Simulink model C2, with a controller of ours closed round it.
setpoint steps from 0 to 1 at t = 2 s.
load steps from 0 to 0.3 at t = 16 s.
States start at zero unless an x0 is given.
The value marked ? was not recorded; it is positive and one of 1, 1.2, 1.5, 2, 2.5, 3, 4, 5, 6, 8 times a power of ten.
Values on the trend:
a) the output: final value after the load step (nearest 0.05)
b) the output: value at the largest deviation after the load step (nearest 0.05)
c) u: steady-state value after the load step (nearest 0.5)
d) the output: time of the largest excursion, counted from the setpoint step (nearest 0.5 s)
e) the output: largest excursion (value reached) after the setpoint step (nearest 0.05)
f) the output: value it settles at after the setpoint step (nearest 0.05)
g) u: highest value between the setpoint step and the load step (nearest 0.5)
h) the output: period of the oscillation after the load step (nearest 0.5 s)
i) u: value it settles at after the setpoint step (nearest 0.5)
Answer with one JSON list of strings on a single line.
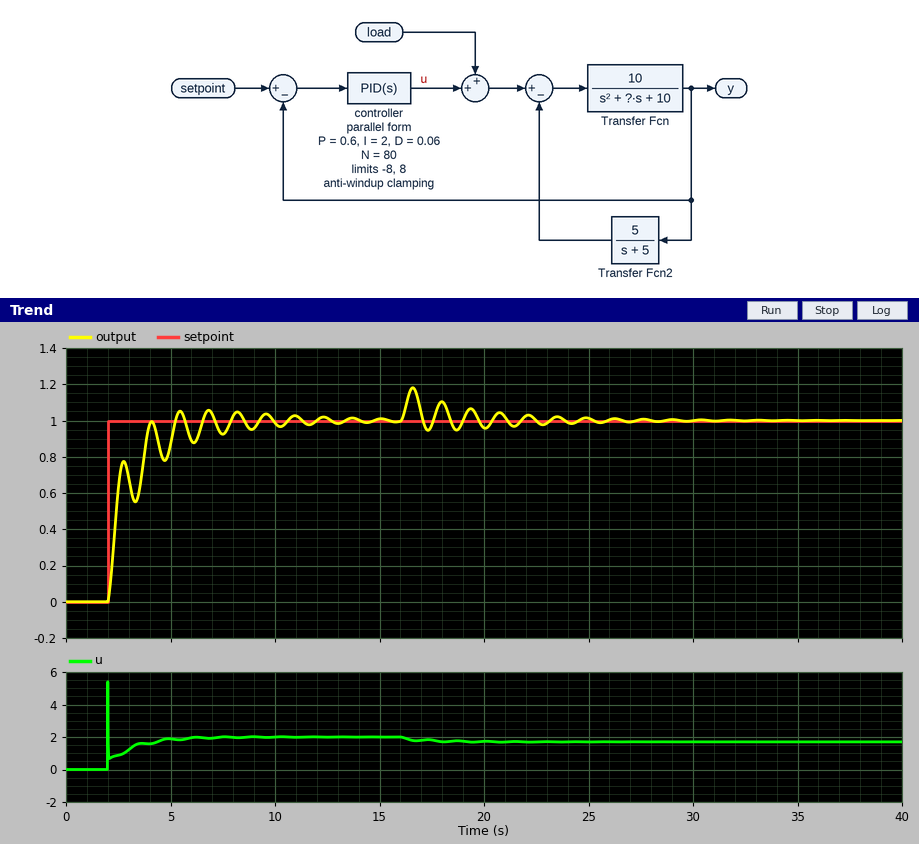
["1.00", "1.20", "1.5", "5.0 s", "1.05", "1.00", "5.5", "1.5 s", "2.0"]
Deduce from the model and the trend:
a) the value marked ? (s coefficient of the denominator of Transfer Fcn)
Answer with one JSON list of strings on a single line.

["2"]
